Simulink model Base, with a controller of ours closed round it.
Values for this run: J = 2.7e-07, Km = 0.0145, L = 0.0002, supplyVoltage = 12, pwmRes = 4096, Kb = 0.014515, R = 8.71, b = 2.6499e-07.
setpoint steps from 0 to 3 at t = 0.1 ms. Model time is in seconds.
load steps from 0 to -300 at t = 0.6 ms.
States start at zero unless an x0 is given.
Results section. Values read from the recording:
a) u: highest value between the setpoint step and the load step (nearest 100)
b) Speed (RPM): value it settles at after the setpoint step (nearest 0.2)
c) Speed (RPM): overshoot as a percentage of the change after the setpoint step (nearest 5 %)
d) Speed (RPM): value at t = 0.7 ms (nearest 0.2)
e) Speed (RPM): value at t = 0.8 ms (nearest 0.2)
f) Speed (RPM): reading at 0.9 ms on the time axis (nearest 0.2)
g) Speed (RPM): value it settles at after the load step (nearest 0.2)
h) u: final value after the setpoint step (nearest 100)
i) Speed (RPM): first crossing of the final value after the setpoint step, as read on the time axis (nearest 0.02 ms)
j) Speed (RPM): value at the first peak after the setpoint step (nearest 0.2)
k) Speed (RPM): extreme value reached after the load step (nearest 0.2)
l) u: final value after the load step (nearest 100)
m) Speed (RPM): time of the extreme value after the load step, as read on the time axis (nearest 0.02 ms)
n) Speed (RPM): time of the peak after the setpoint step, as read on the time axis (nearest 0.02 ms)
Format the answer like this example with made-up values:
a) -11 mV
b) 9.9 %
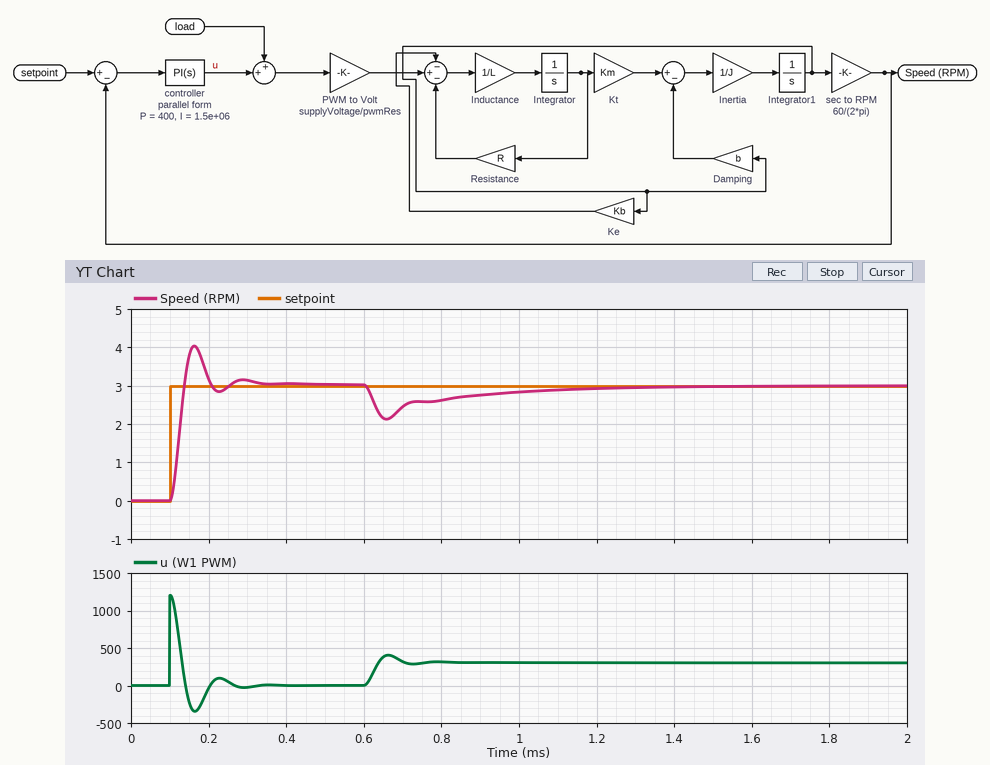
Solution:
a) 1200
b) 3.0
c) 35 %
d) 2.4
e) 2.6
f) 2.8
g) 3.0
h) 0
i) 0.14 ms
j) 4.0
k) 2.2
l) 300
m) 0.66 ms
n) 0.16 ms
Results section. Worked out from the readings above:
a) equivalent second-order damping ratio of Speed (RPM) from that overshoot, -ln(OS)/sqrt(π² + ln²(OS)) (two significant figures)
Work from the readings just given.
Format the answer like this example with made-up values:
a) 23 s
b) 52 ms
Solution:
a) 0.32
